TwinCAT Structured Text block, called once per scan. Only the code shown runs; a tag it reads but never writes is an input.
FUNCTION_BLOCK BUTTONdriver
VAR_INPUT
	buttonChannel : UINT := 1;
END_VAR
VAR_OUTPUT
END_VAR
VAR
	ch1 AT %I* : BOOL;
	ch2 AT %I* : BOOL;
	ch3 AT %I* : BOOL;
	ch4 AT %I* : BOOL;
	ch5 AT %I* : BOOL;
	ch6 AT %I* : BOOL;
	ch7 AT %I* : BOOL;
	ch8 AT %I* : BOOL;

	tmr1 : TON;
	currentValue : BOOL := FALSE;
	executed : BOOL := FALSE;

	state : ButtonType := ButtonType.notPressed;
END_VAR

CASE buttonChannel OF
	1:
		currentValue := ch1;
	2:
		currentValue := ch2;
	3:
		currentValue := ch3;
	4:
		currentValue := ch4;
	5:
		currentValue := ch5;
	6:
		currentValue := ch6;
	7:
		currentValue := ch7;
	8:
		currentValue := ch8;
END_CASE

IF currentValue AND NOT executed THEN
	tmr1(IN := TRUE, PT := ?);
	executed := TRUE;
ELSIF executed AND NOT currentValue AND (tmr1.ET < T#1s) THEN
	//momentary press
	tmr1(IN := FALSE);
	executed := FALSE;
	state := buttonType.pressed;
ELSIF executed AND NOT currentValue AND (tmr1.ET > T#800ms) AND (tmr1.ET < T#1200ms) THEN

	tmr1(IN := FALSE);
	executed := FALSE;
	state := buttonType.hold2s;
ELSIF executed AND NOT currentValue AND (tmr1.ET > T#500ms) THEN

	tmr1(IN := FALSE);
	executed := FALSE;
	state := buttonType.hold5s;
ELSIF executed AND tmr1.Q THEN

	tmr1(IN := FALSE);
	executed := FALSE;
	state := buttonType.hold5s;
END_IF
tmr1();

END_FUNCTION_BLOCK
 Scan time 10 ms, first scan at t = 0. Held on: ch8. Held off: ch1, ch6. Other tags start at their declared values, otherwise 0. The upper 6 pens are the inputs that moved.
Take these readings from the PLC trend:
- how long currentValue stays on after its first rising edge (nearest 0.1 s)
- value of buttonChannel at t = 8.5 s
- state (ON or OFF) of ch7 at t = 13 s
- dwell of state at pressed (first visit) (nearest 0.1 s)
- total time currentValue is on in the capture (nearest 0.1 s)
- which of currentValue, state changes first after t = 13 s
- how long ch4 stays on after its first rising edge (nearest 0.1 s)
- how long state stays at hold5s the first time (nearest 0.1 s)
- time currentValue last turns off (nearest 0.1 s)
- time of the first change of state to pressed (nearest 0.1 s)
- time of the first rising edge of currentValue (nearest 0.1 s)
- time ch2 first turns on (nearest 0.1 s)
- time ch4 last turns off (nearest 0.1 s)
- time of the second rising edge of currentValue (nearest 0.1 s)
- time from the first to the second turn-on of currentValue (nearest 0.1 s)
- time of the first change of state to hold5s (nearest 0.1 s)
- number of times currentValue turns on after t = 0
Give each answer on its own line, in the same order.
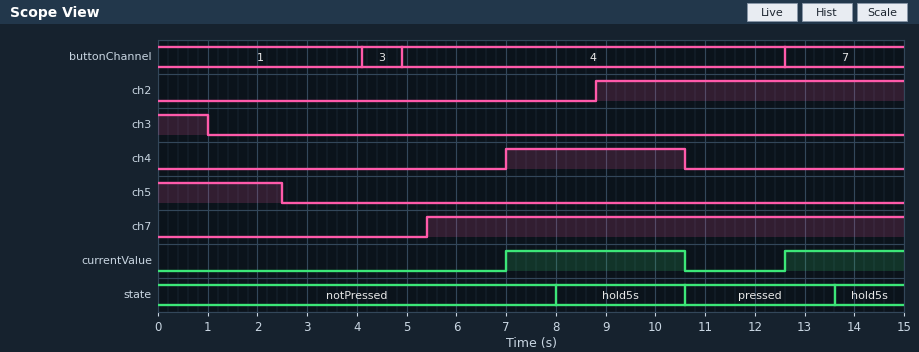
3.6 s
4
ON
3.0 s
6.0 s
state
3.6 s
2.6 s
10.6 s
10.6 s
7.0 s
8.8 s
10.6 s
12.6 s
5.6 s
8.0 s
2
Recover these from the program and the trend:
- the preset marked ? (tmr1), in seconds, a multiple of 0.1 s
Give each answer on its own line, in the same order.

1.0 s
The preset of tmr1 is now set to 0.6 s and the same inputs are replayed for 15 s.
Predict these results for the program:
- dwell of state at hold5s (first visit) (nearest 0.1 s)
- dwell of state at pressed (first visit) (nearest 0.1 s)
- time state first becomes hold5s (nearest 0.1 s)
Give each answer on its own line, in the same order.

3.0 s
2.6 s
7.6 s
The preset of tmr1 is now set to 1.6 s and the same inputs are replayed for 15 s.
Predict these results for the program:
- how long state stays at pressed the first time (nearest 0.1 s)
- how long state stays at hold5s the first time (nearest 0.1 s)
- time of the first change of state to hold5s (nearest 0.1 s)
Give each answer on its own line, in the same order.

3.6 s
2.0 s
8.6 s
